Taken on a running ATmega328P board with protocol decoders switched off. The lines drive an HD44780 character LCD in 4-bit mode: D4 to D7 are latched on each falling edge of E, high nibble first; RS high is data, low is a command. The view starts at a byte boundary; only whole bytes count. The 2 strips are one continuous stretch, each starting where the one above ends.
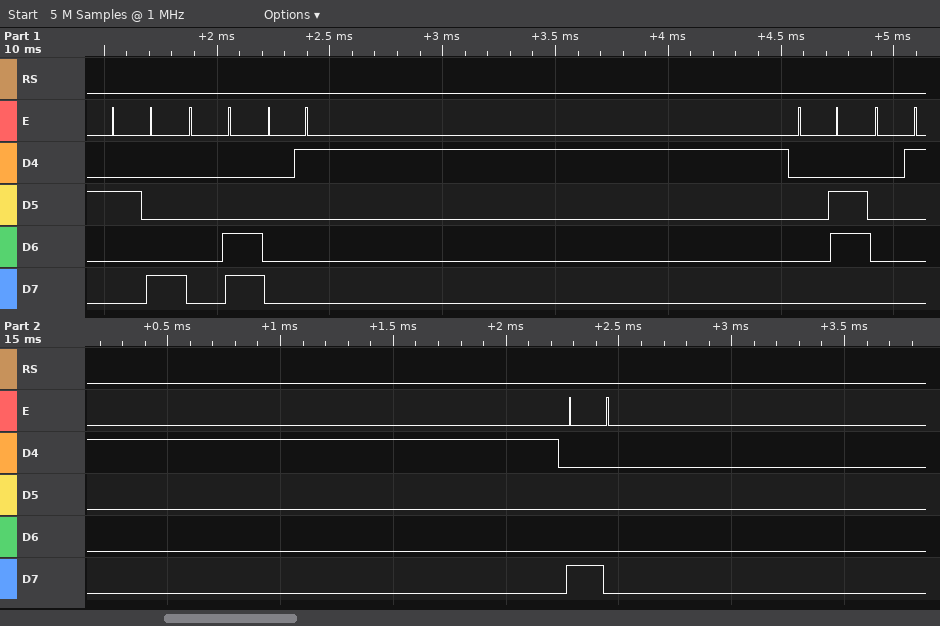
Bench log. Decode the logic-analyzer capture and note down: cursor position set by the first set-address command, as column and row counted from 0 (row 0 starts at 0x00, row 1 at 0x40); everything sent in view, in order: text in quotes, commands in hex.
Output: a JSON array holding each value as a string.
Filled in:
["column 0, row 0", "0x28 0x0C 0x01 0x06 0x01 0x80"]
